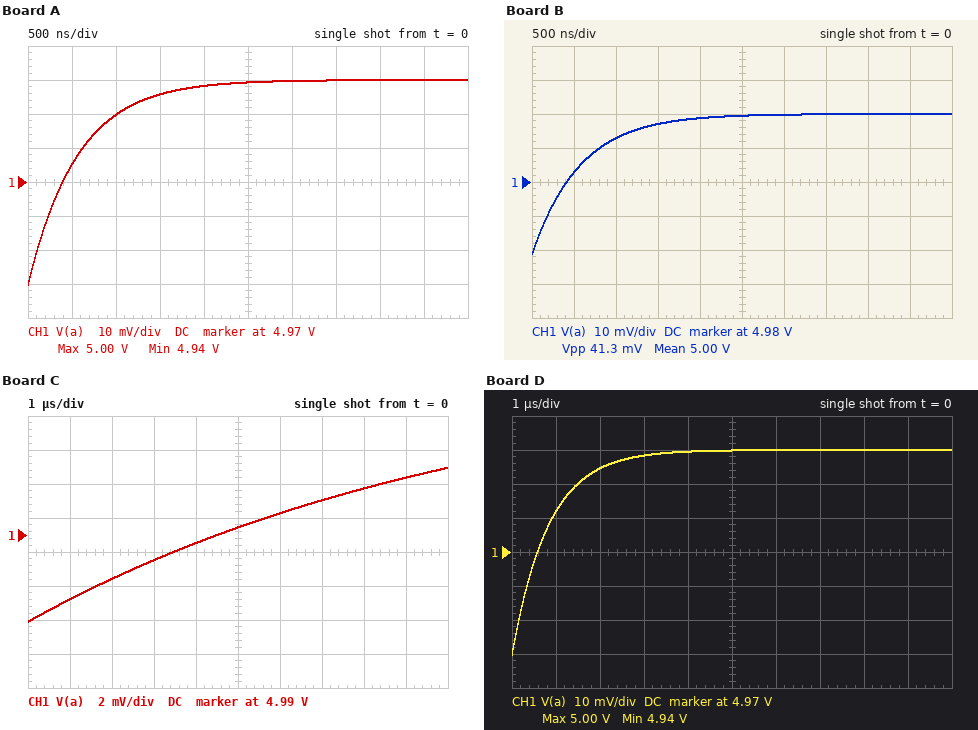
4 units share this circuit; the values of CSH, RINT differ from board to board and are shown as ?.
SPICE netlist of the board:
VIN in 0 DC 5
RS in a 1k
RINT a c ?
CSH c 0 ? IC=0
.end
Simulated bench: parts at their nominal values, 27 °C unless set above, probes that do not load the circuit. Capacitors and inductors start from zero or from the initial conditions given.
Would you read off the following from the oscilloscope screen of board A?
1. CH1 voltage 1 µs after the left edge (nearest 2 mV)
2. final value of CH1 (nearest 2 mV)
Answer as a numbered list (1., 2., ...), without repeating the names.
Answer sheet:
1. 4.990 V
2. 5.000 V
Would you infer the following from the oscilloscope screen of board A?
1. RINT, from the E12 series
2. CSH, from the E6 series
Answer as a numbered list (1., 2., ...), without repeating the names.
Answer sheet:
1. 82 kΩ
2. 6.8 pF
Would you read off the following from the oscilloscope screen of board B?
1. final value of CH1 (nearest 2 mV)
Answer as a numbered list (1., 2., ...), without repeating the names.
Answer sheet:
1. 5.000 V
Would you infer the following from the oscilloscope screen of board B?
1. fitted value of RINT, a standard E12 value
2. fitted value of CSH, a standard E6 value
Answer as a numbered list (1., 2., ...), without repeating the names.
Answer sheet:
1. 120 kΩ
2. 4.7 pF
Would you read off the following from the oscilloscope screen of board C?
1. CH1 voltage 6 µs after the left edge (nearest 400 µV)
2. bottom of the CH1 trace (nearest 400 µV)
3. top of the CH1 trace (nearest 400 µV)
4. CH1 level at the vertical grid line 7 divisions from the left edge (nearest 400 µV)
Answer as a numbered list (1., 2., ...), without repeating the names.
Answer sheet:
1. 4.9912 V
2. 4.9848 V
3. 4.9940 V
4. 4.9920 V
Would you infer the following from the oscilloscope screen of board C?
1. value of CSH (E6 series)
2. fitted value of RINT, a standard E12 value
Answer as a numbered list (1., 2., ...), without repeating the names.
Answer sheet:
1. 33 pF
2. 330 kΩ
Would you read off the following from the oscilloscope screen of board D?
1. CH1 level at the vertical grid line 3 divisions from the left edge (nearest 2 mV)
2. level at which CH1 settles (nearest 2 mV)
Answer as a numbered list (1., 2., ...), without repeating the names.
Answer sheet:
1. 4.998 V
2. 5.000 V
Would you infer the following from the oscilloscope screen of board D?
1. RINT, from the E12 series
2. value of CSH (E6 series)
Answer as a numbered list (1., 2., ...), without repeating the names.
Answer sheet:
1. 82 kΩ
2. 10 pF
